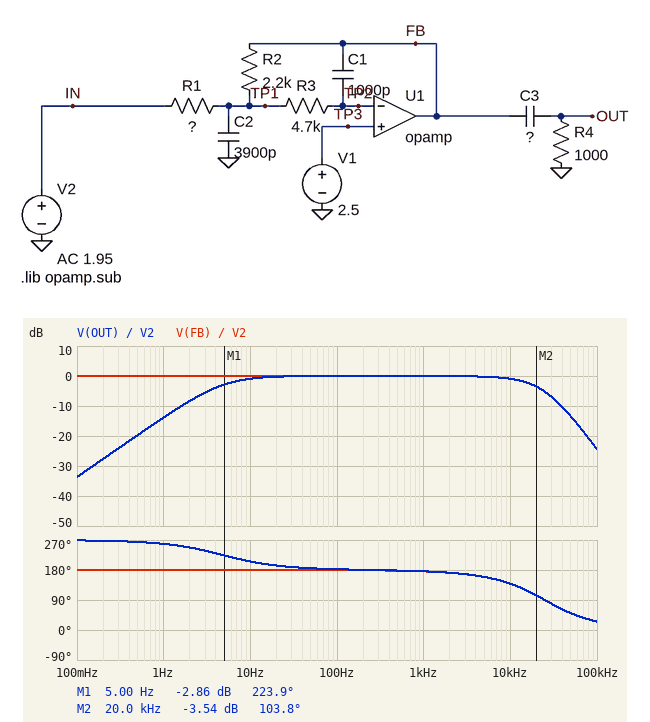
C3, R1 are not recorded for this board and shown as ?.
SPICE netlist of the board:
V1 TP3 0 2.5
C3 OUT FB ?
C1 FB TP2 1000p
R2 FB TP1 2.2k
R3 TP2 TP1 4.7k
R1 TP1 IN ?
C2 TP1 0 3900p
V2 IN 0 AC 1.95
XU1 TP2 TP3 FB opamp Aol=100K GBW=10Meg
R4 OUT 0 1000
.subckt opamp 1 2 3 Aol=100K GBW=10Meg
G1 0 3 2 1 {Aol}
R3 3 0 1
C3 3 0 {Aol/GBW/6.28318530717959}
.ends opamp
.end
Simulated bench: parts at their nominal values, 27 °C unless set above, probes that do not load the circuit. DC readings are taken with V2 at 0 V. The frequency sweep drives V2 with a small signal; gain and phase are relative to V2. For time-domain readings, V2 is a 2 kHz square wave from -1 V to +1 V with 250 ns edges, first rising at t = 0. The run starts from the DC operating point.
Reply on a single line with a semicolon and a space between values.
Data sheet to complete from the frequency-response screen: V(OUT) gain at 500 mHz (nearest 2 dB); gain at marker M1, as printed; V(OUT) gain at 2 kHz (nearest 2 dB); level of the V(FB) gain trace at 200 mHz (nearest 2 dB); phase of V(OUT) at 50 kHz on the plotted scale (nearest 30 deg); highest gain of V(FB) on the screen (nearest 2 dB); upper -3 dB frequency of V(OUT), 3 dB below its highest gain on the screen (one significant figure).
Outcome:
-20 dB; -2.86 dB; 0 dB; 0 dB; 60 deg; 0 dB; 20 kHz
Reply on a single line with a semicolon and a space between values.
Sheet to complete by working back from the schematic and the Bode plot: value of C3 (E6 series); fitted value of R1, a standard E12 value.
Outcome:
33 µF; 2.2 kΩ
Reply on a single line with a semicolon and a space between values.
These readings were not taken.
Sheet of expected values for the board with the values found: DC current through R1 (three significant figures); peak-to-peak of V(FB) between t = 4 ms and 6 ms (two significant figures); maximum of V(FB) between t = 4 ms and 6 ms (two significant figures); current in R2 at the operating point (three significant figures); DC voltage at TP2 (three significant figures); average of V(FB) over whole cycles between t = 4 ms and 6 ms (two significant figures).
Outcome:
1.14 mA; 2.0 V; 6.0 V; 1.14 mA; 2.50 V; 5.0 V
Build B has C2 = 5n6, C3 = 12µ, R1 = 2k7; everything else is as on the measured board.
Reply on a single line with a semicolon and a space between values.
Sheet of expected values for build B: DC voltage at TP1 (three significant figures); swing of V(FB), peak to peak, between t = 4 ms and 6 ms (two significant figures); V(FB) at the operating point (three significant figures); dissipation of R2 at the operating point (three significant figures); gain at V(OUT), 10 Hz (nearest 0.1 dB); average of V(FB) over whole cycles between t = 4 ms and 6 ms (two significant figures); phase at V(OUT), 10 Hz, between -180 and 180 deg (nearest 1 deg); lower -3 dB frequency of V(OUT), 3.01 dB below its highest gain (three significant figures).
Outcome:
2.50 V; 1.8 V; 4.54 V; 1.89 mW; -6.2 dB; 4.5 V; -127 deg; 13.3 Hz
